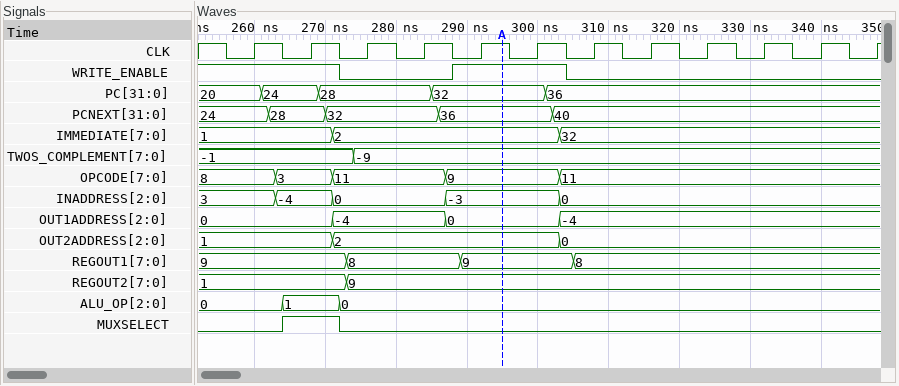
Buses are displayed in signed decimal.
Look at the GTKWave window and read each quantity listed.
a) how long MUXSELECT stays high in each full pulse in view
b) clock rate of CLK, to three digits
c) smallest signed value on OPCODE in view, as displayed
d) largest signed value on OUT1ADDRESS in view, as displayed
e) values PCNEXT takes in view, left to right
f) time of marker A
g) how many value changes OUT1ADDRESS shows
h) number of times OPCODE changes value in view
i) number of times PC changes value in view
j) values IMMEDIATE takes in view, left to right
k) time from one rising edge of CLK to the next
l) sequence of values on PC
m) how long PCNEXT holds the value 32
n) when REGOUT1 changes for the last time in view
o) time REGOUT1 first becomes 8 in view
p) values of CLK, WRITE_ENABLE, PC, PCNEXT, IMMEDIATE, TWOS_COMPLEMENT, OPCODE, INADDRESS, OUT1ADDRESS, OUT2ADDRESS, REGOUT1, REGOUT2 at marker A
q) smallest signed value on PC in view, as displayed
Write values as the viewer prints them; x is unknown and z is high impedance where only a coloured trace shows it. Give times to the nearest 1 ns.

8 ns
125 MHz
3
0
24, 28, 32, 36, 40
295 ns
3
4
4
1, 2, 32
8 ns
20, 24, 28, 32, 36
16 ns
305 ns
273 ns
CLK=1, WRITE_ENABLE=1, PC=32, PCNEXT=36, IMMEDIATE=2, TWOS_COMPLEMENT=-9, OPCODE=9, INADDRESS=-3, OUT1ADDRESS=0, OUT2ADDRESS=2, REGOUT1=9, REGOUT2=9
20
